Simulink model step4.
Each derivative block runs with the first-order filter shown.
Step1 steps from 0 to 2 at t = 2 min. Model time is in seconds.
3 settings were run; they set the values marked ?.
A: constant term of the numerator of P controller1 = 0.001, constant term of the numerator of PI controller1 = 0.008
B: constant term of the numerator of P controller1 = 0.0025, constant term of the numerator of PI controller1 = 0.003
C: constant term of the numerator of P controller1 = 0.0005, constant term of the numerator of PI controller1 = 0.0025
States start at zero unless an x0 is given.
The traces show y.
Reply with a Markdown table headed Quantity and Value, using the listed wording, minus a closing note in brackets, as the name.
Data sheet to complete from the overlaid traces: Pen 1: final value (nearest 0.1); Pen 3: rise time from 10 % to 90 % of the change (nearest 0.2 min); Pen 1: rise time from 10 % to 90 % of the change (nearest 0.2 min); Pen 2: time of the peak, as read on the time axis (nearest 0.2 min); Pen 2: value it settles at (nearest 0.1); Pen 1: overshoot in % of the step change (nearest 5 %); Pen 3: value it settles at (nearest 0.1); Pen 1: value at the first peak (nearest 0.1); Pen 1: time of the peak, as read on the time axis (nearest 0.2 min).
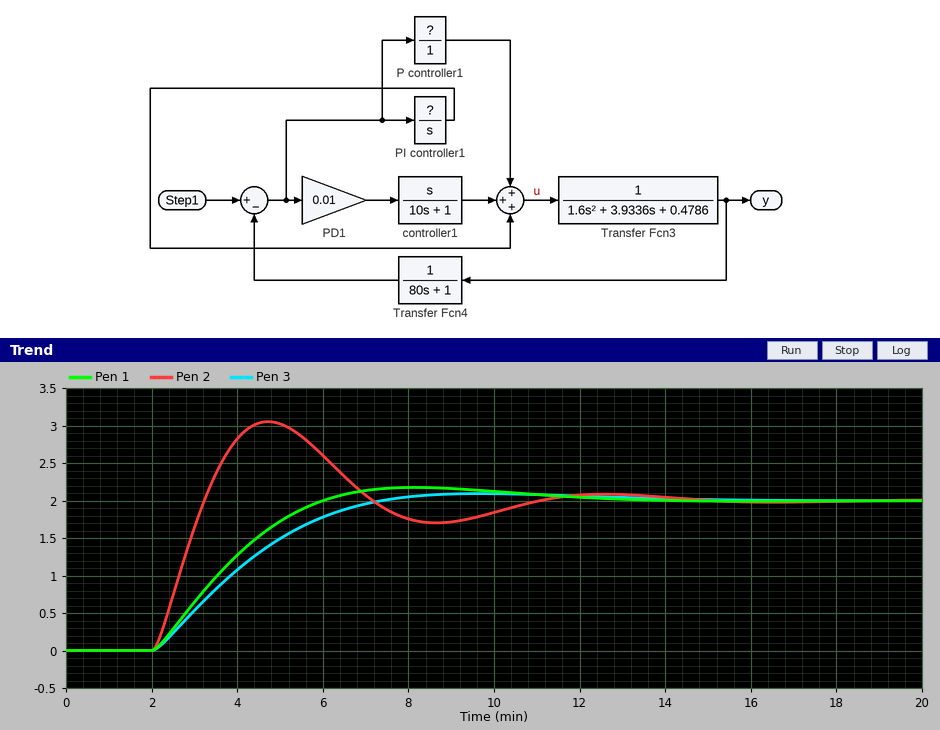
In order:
| Quantity | Value |
|---|---|
| Pen 1: final value | 2.0 |
| Pen 3: rise time from 10 % to 90 % of the change | 3.6 min |
| Pen 1: rise time from 10 % to 90 % of the change | 2.8 min |
| Pen 2: time of the peak, as read on the time axis | 4.8 min |
| Pen 2: value it settles at | 2.0 |
| Pen 1: overshoot in % of the step change | 10 % |
| Pen 3: value it settles at | 2.0 |
| Pen 1: value at the first peak | 2.2 |
| Pen 1: time of the peak, as read on the time axis | 8.2 min |
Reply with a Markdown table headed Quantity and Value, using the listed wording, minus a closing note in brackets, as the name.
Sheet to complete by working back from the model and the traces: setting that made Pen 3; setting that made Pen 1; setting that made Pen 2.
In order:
| Quantity | Value |
|---|---|
| setting that made Pen 3 | C |
| setting that made Pen 1 | B |
| setting that made Pen 2 | A |
